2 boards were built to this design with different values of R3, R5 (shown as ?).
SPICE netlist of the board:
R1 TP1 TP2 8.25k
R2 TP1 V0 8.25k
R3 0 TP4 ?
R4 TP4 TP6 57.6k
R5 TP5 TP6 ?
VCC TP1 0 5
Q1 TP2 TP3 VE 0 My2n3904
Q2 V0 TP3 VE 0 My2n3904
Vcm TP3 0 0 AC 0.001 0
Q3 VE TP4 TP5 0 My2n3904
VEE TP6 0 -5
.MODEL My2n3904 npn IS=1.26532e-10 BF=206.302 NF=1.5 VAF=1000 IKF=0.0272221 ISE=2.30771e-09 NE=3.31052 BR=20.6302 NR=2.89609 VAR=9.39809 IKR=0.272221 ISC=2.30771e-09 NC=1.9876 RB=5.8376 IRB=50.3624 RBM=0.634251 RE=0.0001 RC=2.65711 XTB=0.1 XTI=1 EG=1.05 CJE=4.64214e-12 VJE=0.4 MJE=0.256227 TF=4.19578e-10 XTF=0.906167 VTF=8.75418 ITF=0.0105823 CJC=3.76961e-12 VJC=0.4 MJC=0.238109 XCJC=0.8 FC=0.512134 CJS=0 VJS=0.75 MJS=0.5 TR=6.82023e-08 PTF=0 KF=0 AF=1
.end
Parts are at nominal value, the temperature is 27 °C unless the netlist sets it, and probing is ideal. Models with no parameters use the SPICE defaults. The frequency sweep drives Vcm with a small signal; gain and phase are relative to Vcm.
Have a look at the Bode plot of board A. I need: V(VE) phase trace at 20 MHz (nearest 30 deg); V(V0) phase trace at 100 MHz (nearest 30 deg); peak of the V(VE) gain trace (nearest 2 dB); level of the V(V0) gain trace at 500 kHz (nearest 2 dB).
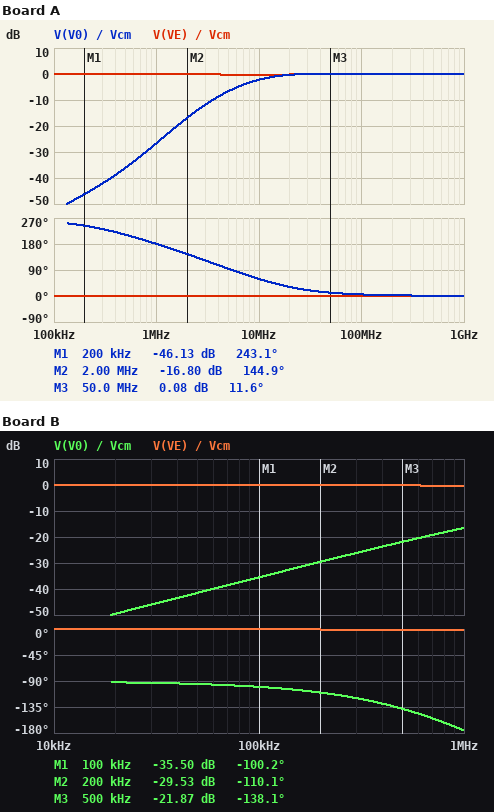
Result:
0 deg
0 deg
0 dB
-36 dB
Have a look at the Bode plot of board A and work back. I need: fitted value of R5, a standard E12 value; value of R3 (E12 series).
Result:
22 kΩ
33 kΩ
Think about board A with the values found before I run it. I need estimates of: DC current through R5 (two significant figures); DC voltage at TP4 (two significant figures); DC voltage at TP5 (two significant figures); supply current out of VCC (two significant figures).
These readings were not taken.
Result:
120 µA
-1.9 V
-2.4 V
110 µA
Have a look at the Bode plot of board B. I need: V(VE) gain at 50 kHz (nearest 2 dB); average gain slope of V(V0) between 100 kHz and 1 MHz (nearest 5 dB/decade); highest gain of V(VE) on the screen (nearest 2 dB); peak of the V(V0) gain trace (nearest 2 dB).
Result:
0 dB
20 dB/decade
0 dB
-16 dB
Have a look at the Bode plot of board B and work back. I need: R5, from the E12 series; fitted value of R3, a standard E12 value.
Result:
10 kΩ
270 kΩ
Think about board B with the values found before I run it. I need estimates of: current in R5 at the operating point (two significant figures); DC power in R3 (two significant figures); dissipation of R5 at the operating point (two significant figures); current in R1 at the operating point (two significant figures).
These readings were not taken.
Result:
35 µA
64 µW
12 µW
17 µA
